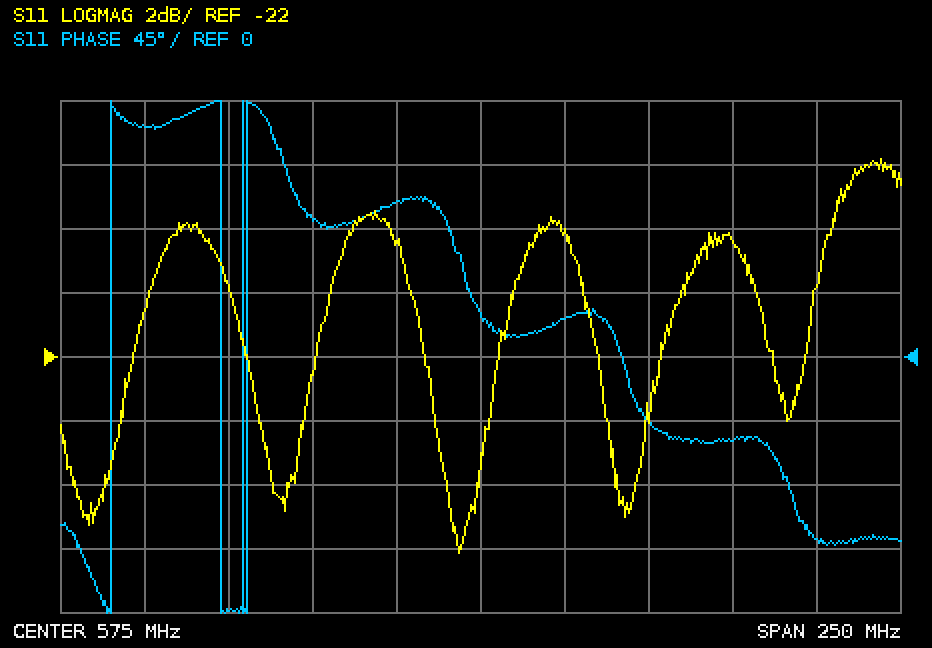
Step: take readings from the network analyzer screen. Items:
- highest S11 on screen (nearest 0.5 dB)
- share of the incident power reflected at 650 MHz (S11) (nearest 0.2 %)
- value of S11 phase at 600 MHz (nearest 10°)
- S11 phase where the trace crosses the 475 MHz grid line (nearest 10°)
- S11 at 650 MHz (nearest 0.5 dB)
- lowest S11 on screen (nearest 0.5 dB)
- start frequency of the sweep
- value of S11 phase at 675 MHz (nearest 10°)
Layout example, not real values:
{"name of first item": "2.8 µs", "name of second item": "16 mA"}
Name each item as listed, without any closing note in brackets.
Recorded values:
{"highest S11 on screen": "-16.0 dB", "share of the incident power reflected at 650 MHz (S11)": "1.4 %", "value of S11 phase at 600 MHz": "30°", "S11 phase where the trace crosses the 475 MHz grid line": "160°", "S11 at 650 MHz": "-18.5 dB", "lowest S11 on screen": "-28.0 dB", "start frequency of the sweep": "450 MHz", "value of S11 phase at 675 MHz": "-130°"}
